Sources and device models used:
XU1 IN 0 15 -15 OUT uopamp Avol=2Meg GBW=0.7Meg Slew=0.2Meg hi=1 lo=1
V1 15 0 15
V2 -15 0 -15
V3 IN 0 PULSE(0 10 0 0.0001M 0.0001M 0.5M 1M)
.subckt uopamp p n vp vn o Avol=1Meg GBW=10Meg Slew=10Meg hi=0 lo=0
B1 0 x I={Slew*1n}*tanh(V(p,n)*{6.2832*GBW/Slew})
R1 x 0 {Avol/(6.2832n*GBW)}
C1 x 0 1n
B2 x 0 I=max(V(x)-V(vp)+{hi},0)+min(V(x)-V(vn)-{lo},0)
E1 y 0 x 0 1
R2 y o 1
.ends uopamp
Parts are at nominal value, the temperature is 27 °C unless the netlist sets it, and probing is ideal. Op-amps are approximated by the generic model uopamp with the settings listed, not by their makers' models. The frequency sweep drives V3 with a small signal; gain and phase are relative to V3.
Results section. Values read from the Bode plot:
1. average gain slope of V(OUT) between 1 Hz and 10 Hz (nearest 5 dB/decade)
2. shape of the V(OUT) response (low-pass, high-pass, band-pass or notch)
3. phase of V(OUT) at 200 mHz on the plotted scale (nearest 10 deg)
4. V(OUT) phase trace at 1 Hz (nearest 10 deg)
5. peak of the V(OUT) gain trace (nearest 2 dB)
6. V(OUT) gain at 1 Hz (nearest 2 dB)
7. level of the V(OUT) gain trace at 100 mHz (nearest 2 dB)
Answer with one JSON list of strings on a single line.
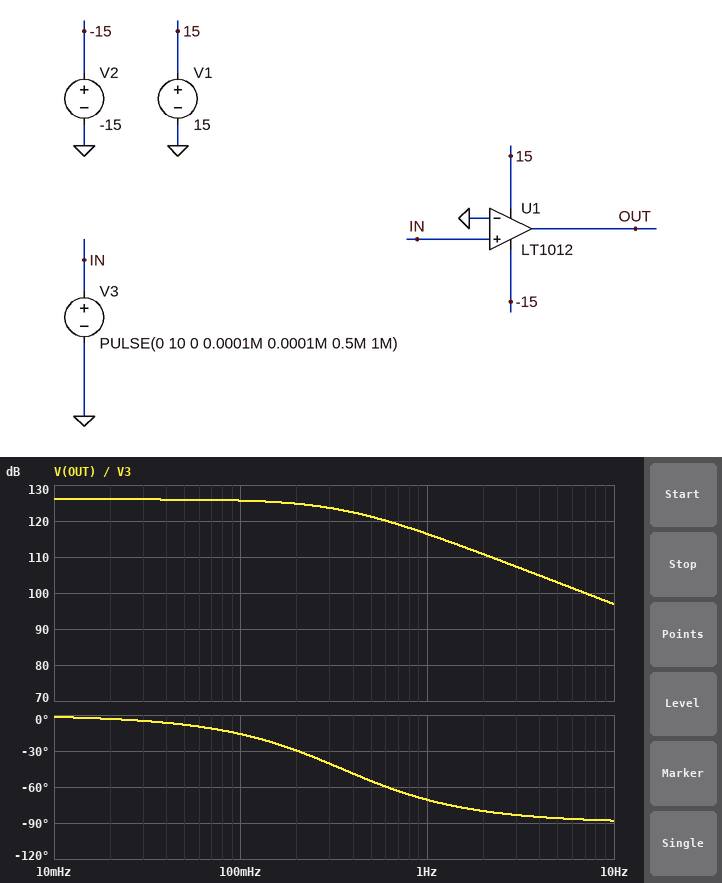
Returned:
["-20 dB/decade", "low-pass", "-30 deg", "-70 deg", "126 dB", "116 dB", "126 dB"]
